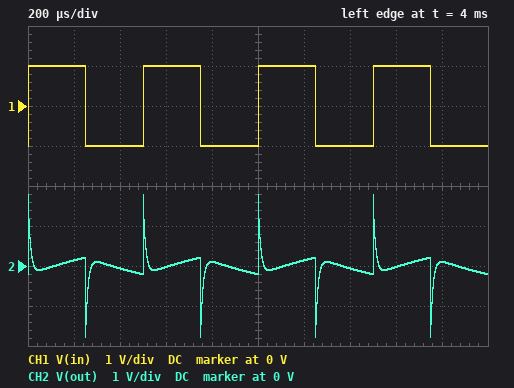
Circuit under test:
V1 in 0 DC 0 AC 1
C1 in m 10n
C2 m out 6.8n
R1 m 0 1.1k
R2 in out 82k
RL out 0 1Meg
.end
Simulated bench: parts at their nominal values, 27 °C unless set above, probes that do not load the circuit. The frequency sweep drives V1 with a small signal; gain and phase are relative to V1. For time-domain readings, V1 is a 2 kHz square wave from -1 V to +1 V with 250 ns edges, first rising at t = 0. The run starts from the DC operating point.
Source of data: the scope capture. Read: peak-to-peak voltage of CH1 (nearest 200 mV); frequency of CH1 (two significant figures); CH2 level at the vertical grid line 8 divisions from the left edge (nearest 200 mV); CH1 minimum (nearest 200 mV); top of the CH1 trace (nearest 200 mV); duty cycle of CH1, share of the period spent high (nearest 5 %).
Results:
2.0 V
2.0 kHz
0 V
-1.0 V
1.0 V
50 %
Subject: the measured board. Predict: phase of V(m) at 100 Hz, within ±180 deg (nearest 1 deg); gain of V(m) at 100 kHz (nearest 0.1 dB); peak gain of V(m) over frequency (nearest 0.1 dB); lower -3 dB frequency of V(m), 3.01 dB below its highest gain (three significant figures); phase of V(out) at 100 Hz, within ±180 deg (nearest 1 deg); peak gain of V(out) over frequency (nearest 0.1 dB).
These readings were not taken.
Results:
83 deg
-0.1 dB
0 dB
14.7 kHz
-18 deg
0 dB
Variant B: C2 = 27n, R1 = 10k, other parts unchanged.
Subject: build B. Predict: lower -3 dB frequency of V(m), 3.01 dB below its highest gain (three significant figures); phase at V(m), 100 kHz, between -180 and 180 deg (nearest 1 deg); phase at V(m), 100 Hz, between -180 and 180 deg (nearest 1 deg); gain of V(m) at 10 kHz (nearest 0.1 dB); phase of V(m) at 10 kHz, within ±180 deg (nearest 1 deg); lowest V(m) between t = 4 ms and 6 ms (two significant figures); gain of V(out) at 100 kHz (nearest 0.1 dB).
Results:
1.77 kHz
1 deg
51 deg
-0.1 dB
9 deg
-1.8 V
0 dB
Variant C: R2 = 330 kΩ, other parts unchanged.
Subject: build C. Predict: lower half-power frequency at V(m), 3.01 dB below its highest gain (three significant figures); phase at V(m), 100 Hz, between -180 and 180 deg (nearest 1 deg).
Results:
14.5 kHz
78 deg
